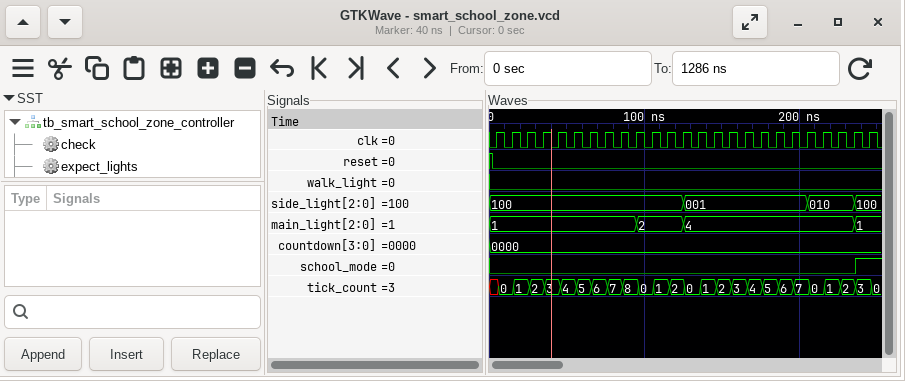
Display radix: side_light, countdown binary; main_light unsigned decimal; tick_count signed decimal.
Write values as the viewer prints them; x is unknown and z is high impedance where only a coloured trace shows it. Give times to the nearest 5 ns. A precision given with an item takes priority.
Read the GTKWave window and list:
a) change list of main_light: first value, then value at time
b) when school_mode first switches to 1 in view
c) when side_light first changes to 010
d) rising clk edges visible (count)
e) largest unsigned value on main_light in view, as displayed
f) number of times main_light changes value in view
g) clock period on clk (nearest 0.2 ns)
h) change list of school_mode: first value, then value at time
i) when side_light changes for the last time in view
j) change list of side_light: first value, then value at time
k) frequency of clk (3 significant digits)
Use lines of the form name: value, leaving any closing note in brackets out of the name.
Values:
change list of main_light: first value, then value at time: 1, 2 at 95 ns, 4 at 125 ns, 1 at 235 ns
when school_mode first switches to 1 in view: 235 ns
when side_light first changes to 010: 205 ns
rising clk edges visible: 25
largest unsigned value on main_light in view, as displayed: 4
number of times main_light changes value in view: 3
clock period on clk: 10 ns
change list of school_mode: first value, then value at time: 0, 1 at 235 ns
when side_light changes for the last time in view: 235 ns
change list of side_light: first value, then value at time: 100, 001 at 125 ns, 010 at 205 ns, 100 at 235 ns
frequency of clk: 100 MHz
